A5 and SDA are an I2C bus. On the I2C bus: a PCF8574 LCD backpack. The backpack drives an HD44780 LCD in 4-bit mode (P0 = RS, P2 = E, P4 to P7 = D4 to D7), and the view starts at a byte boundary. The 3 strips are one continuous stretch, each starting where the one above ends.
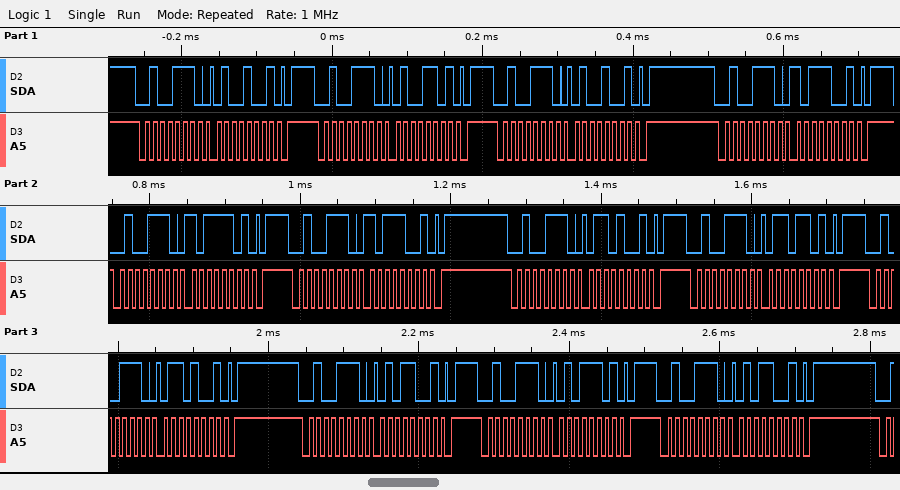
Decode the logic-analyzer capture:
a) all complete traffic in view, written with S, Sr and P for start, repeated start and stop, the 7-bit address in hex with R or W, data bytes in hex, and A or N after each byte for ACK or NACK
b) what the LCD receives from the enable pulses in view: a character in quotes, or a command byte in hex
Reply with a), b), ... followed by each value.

a) S 27W A 49 A P S 27W A 4D A P S 27W A 49 A P S 27W A B9 A P S 27W A BD A P S 27W A B9 A P S 27W A 69 A P S 27W A 6D A P S 27W A 69 A P S 27W A 59 A P S 27W A 5D A P S 27W A 59 A P
b) 'K' 'e'
